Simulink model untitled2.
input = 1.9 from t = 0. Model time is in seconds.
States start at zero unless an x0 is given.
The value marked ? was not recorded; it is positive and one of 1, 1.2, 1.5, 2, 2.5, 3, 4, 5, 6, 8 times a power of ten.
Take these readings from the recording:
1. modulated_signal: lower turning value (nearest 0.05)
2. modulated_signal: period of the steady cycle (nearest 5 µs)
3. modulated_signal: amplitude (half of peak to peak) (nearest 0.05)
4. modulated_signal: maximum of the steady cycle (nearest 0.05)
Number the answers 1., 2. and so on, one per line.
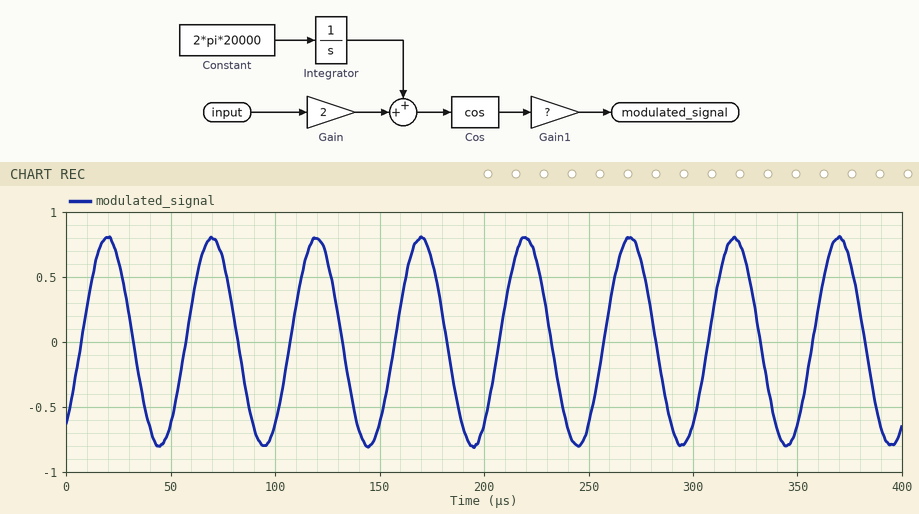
1. -0.80
2. 50 µs
3. 0.80
4. 0.80
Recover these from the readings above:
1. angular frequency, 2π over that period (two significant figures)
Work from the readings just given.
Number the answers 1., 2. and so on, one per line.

1. 0.13 rad/µs
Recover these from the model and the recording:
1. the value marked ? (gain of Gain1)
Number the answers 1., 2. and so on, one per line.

1. 0.8
